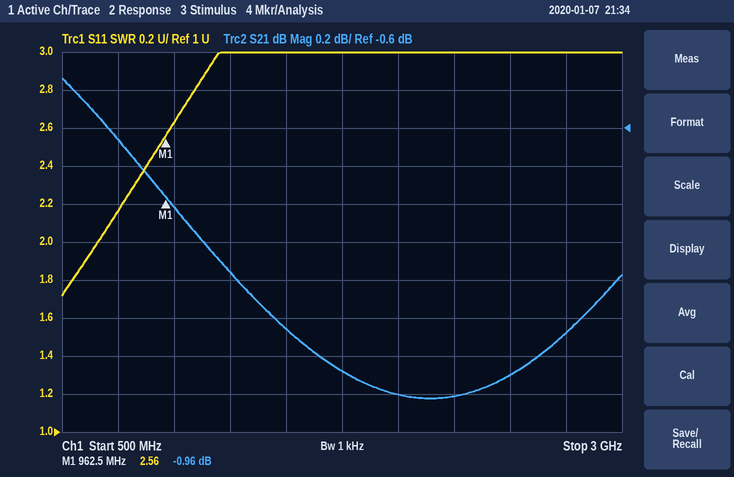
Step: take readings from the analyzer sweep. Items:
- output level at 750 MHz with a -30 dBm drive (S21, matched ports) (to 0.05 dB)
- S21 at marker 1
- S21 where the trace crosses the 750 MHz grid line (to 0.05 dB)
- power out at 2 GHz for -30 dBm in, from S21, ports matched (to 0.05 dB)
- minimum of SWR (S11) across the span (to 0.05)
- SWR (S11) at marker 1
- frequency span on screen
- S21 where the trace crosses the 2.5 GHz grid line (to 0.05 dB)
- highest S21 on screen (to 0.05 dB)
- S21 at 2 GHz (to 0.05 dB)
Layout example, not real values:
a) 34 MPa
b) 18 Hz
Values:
a) -30.65 dBm
b) -0.96 dB
c) -0.65 dB
d) -32.00 dBm
e) 1.70
f) 2.56
g) 2.5 GHz
h) -1.90 dB
i) -0.35 dB
j) -2.00 dB
